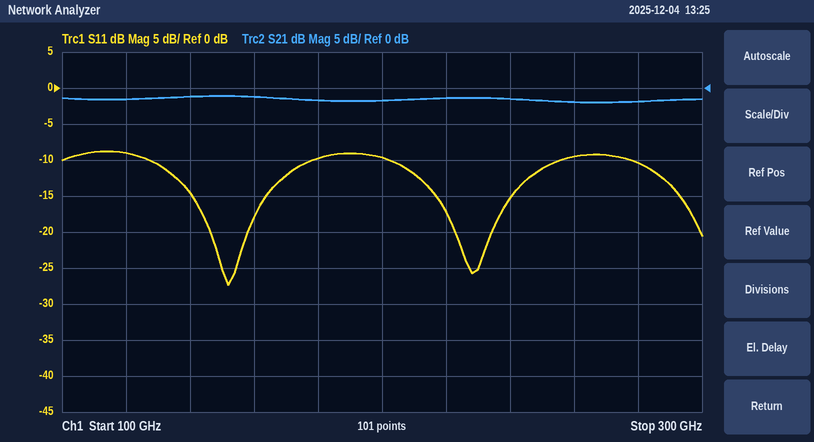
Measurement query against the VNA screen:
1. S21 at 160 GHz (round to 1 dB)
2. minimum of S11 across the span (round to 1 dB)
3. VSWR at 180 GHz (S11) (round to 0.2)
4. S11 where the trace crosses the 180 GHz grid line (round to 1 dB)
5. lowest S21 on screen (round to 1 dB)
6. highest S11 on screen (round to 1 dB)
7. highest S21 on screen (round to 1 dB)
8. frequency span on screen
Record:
-1 dB
-27 dB
2.0
-10 dB
-2 dB
-9 dB
-1 dB
200 GHz
